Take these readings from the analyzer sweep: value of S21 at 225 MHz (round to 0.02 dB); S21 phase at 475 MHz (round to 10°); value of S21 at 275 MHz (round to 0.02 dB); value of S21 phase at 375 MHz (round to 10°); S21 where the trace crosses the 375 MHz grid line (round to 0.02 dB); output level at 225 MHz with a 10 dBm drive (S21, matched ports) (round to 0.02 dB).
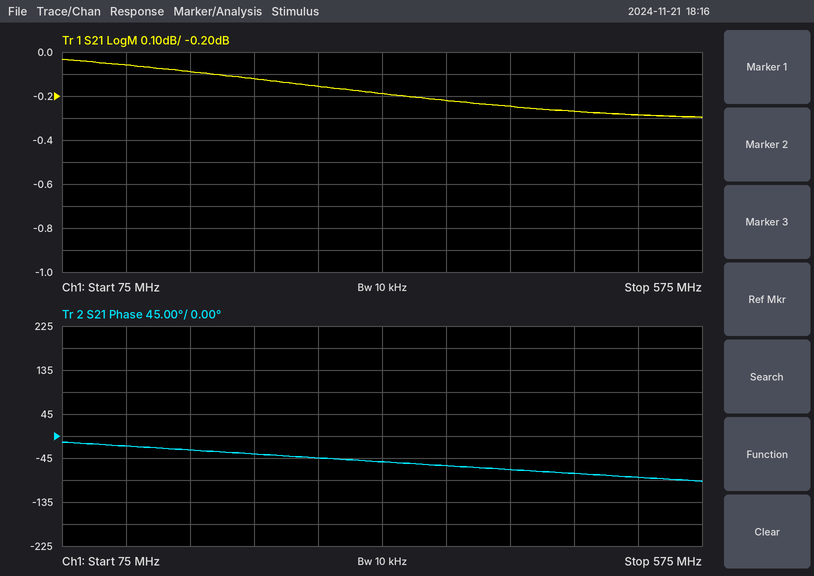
-0.12 dB
-80°
-0.16 dB
-60°
-0.22 dB
9.88 dBm
